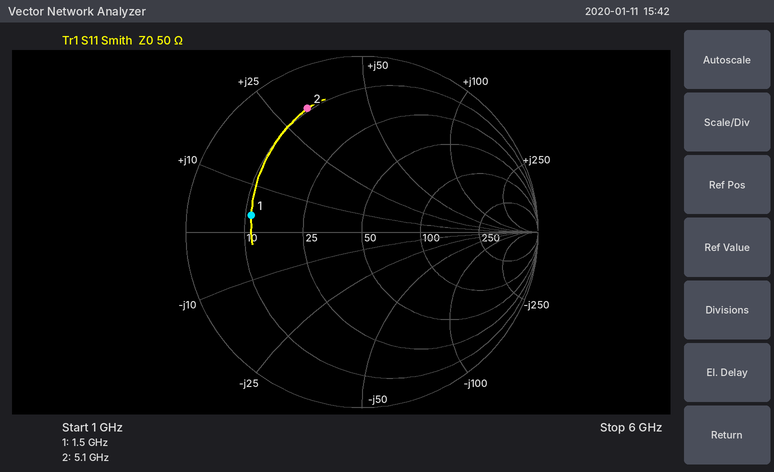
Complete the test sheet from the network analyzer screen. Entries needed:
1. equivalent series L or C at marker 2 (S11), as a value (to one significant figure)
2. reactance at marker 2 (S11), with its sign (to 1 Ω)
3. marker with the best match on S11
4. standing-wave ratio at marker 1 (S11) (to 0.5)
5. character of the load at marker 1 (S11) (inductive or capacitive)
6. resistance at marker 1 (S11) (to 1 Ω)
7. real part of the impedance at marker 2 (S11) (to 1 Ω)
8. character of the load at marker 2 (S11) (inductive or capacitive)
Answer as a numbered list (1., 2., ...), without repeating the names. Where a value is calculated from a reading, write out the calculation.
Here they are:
1. L = 32 Ω/(2π × 5.1 GHz) ≈ 1.0 nH
2. +32 Ω
3. marker 1
4. 4.5
5. inductive
6. 11 Ω
7. 9 Ω
8. inductive
